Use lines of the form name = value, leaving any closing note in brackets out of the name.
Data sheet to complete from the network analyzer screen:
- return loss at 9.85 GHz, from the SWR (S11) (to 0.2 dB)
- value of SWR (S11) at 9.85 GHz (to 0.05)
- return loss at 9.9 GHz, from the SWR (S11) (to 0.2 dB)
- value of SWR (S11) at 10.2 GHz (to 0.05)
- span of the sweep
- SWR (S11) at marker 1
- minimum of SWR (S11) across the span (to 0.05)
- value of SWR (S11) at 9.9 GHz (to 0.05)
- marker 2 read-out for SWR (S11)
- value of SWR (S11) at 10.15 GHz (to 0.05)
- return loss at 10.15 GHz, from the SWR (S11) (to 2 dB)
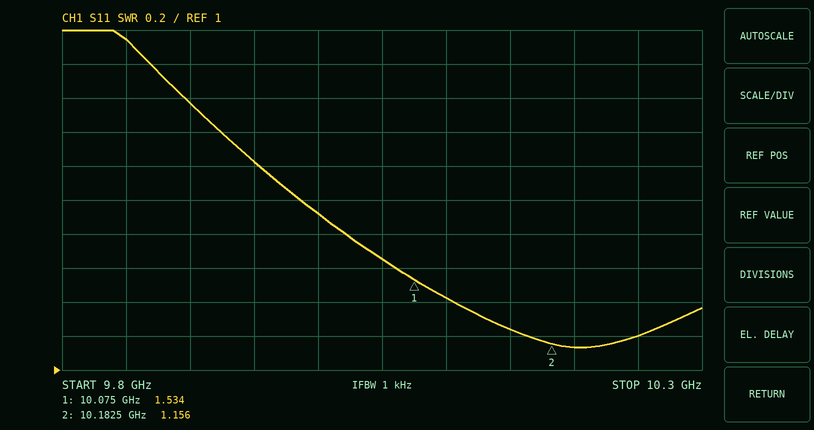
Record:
return loss at 9.85 GHz, from the SWR (S11) = 6.2 dB
value of SWR (S11) at 9.85 GHz = 2.95
return loss at 9.9 GHz, from the SWR (S11) = 7.2 dB
value of SWR (S11) at 10.2 GHz = 1.15
span of the sweep = 500 MHz
SWR (S11) at marker 1 = 1.534
minimum of SWR (S11) across the span = 1.15
value of SWR (S11) at 9.9 GHz = 2.55
marker 2 read-out for SWR = 1.156
value of SWR (S11) at 10.15 GHz = 1.25
return loss at 10.15 GHz, from the SWR (S11) = 20 dB
